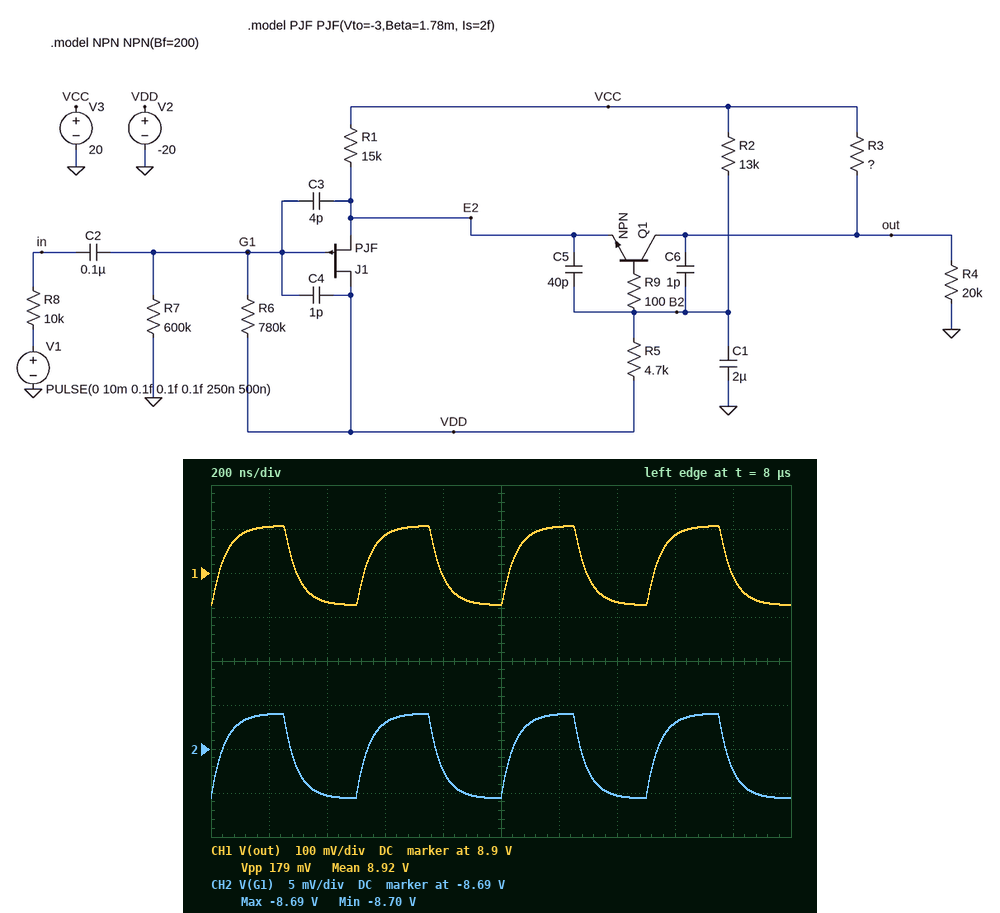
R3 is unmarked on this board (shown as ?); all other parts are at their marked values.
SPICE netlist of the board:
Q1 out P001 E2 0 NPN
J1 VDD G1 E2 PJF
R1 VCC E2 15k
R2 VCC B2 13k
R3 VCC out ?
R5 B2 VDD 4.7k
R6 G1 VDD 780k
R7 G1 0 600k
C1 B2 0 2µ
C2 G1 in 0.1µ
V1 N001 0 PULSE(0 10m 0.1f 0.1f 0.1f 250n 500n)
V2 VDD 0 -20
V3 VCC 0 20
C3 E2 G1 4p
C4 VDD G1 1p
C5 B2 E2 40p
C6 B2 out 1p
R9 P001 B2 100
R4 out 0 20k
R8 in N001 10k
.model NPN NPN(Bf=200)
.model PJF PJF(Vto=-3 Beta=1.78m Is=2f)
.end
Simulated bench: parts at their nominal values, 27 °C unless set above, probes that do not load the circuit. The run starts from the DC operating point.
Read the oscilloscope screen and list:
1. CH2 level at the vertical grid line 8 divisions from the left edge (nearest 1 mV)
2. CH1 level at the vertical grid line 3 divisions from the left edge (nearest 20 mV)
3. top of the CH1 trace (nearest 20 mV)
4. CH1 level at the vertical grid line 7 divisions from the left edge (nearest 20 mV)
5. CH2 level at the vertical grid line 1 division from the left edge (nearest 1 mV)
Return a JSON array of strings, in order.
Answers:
["-8.687 V", "8.98 V", "9.00 V", "8.84 V", "-8.686 V"]
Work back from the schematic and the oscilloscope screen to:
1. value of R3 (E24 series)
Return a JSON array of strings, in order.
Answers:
["4.7 kΩ"]
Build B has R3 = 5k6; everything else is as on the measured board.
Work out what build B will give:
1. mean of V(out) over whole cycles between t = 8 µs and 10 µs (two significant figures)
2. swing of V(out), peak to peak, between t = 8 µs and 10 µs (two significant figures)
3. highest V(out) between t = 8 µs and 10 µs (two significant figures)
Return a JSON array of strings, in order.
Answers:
["7.3 V", "210 mV", "7.4 V"]
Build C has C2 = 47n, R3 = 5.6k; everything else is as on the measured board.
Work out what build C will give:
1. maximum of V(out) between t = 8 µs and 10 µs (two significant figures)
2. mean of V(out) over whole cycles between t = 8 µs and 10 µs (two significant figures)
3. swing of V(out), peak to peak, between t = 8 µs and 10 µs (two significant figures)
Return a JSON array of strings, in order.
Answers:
["7.4 V", "7.3 V", "210 mV"]
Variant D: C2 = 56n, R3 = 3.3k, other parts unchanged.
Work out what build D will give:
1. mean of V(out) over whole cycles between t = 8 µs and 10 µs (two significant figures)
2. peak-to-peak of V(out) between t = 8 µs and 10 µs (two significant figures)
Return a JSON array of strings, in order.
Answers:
["12 V", "130 mV"]
